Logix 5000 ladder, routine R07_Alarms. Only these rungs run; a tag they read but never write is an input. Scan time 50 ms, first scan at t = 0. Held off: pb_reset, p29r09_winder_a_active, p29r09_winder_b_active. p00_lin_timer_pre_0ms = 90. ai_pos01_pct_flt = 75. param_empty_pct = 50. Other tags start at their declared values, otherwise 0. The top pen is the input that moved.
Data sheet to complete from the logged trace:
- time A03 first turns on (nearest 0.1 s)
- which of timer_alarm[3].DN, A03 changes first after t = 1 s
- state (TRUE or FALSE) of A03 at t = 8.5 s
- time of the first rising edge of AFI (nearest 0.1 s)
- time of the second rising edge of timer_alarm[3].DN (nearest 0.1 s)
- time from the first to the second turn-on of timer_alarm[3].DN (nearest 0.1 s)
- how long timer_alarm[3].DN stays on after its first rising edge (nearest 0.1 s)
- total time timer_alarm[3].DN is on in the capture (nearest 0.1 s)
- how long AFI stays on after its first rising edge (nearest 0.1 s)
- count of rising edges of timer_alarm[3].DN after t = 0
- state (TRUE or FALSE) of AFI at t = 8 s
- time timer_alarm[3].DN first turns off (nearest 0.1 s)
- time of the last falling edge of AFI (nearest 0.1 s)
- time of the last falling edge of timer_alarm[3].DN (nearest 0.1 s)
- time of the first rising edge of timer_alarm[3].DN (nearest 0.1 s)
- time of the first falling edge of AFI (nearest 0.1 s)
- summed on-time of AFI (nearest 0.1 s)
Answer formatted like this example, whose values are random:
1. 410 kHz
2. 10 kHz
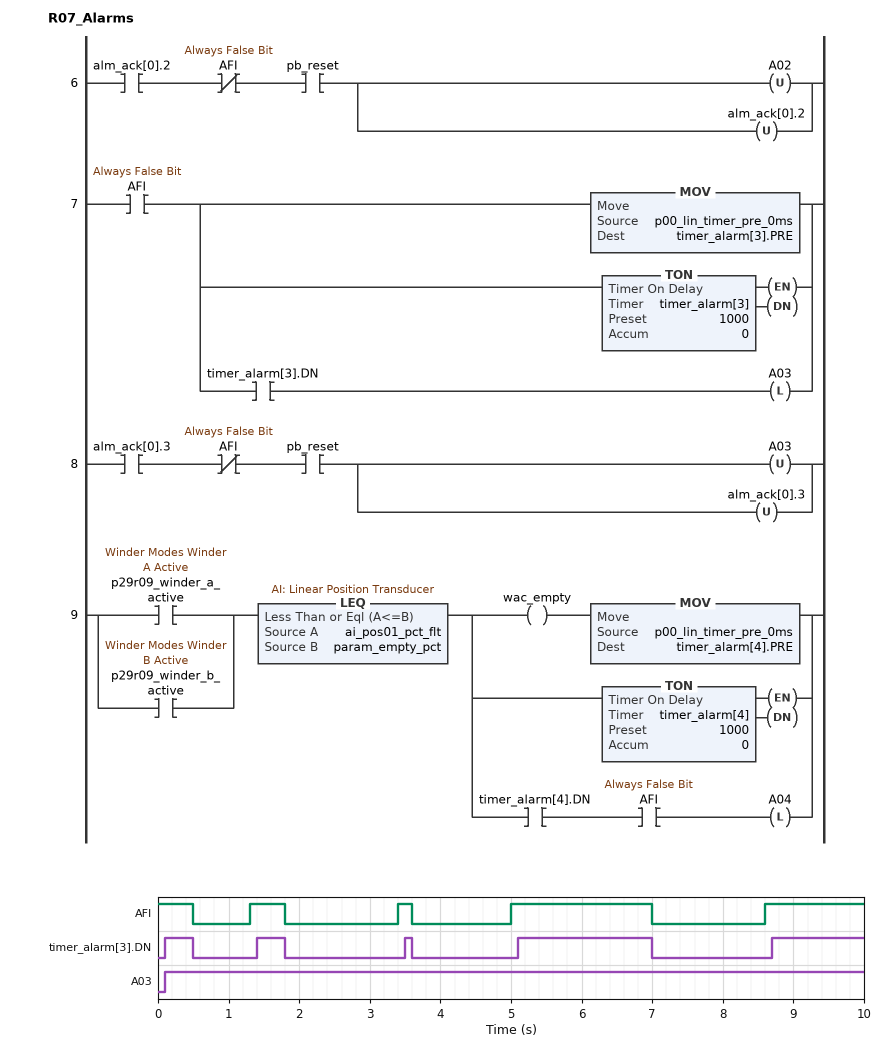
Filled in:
1. 0.1 s
2. timer_alarm[3].DN
3. TRUE
4. 1.3 s
5. 1.4 s
6. 1.3 s
7. 0.4 s
8. 4.1 s
9. 0.5 s
10. 5
11. FALSE
12. 0.5 s
13. 7.0 s
14. 7.0 s
15. 0.1 s
16. 0.5 s
17. 4.6 s
